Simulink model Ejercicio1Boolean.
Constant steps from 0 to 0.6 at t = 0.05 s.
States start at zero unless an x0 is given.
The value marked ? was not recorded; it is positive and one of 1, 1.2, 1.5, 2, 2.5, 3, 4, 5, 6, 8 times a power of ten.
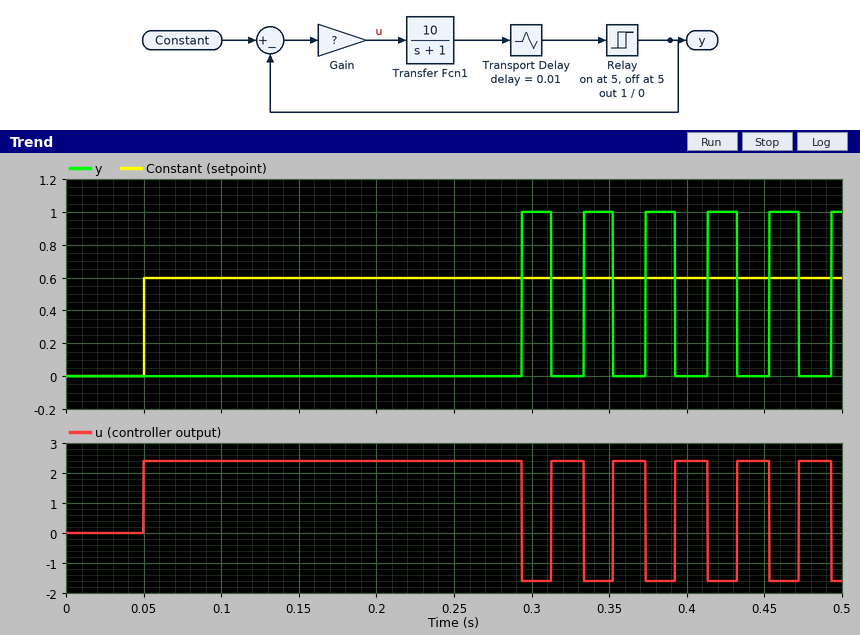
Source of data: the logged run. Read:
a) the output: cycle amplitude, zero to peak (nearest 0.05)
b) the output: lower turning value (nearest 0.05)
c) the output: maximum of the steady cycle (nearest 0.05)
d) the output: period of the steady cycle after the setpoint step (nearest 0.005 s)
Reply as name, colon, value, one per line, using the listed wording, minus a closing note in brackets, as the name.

the output: cycle amplitude, zero to peak: 0.50
the output: lower turning value: 0.00
the output: maximum of the steady cycle: 1.00
the output: period of the steady cycle after the setpoint step: 0.040 s
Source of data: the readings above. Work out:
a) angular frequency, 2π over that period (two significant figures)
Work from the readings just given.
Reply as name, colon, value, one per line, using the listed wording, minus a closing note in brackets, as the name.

angular frequency, 2π over that period: 160 rad/s
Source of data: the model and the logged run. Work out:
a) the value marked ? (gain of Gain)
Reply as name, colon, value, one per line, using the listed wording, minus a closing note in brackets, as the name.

the value marked ?: 4
